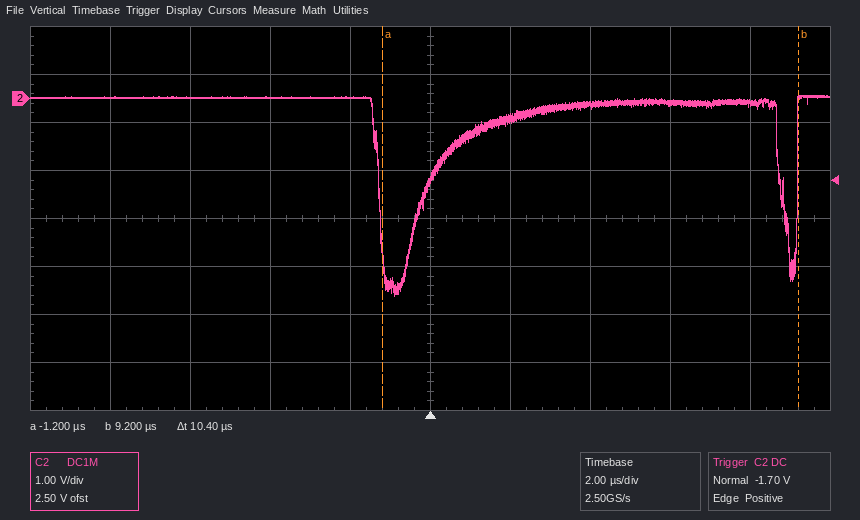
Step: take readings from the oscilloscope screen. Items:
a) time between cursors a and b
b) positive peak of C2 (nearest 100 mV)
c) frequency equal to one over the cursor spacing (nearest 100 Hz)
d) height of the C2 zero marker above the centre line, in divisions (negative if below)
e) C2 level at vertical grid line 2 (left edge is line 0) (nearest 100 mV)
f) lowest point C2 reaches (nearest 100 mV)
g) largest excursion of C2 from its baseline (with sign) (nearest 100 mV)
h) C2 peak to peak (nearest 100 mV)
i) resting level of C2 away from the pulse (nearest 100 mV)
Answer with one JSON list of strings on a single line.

["10.4 µs", "100 mV", "96.2 kHz", "+2.5 div", "0.0 V", "-4.1 V", "-4.1 V", "4.2 V", "0.0 V"]
